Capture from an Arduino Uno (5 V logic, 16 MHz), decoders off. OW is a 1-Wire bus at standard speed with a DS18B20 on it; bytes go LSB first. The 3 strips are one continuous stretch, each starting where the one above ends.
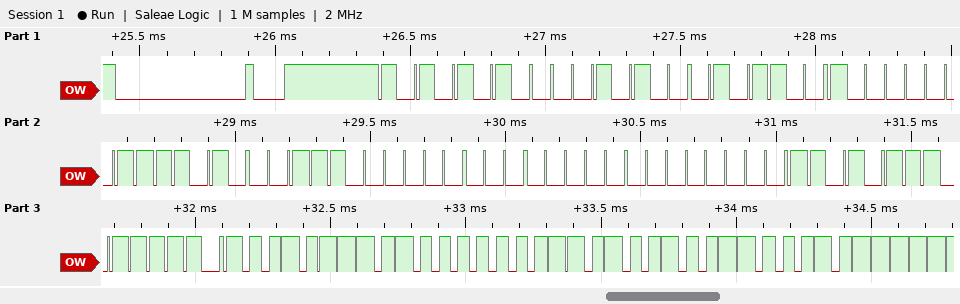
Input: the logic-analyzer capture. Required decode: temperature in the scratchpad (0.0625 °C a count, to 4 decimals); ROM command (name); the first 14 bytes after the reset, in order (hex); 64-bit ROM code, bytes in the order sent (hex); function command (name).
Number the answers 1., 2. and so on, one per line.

1. 23.2500 °C
2. Match ROM
3. 55 28 9A C0 8B 03 00 00 EB BE 74 01 4B 46
4. 28 9A C0 8B 03 00 00 EB
5. Read Scratchpad
